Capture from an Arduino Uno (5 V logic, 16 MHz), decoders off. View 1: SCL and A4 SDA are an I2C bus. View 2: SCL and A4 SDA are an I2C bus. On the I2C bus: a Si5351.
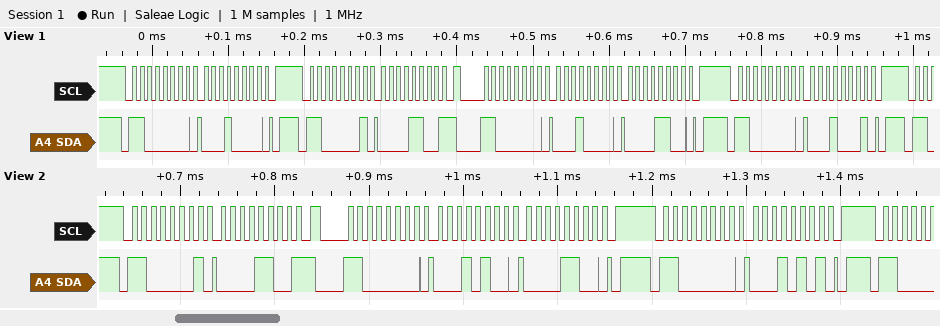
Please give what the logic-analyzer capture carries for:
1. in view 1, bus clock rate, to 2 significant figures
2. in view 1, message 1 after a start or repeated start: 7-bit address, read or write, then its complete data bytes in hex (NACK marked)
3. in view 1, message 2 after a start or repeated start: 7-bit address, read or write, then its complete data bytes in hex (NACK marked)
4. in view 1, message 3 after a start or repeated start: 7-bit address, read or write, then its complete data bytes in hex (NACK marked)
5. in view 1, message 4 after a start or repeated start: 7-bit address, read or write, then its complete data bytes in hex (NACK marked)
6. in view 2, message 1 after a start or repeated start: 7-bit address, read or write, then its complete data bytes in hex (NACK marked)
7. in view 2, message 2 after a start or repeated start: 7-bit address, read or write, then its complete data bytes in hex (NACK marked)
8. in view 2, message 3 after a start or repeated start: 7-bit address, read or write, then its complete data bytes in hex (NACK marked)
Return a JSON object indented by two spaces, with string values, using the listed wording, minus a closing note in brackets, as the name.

{
  "in view 1, bus clock rate, to 2 significant figures": "100 kHz",
  "in view 1, message 1 after a start or repeated start: 7-bit address, read or write, then its complete data bytes in hex": "0x60 write: 10",
  "in view 1, message 2 after a start or repeated start: 7-bit address, read or write, then its complete data bytes in hex": "0x60 read: 0C NACK",
  "in view 1, message 3 after a start or repeated start: 7-bit address, read or write, then its complete data bytes in hex": "0x60 write: 10 0C",
  "in view 1, message 4 after a start or repeated start: 7-bit address, read or write, then its complete data bytes in hex": "0x60 write: 11",
  "in view 2, message 1 after a start or repeated start: 7-bit address, read or write, then its complete data bytes in hex": "0x60 read: 0C NACK",
  "in view 2, message 2 after a start or repeated start: 7-bit address, read or write, then its complete data bytes in hex": "0x60 write: 14 0C",
  "in view 2, message 3 after a start or repeated start: 7-bit address, read or write, then its complete data bytes in hex": "0x60 write: 15"
}
